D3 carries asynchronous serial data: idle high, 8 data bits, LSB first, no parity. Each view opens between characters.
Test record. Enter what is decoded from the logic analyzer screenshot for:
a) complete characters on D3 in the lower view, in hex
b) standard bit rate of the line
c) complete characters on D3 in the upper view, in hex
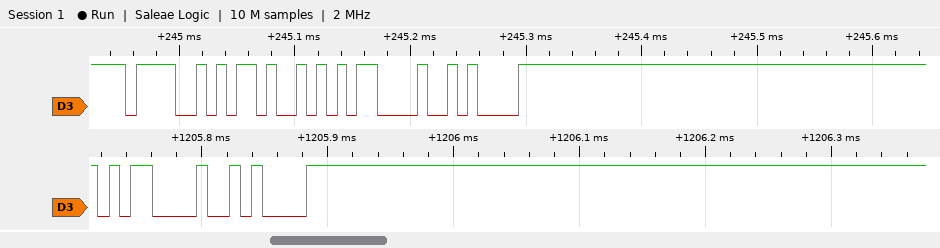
0D, 0A
115200 baud
4F, 4B, 0D, 0A
